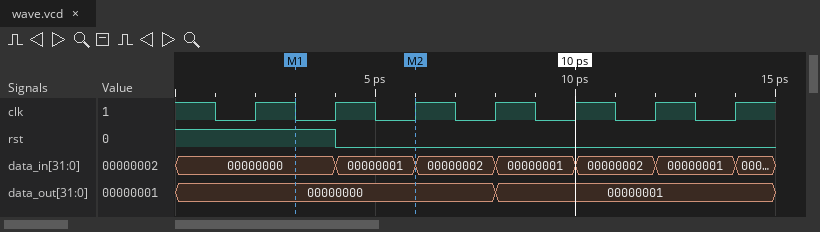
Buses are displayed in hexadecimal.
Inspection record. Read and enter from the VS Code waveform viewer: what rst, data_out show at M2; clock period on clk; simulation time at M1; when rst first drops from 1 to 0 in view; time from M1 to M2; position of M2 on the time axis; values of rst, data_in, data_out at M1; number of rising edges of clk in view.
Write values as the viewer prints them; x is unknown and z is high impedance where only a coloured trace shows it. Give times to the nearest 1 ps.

rst=0, data_out=00000000
2 ps
3 ps
4 ps
3 ps
6 ps
rst=1, data_in=00000000, data_out=00000000
7
